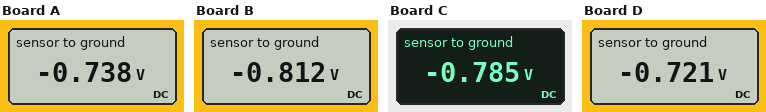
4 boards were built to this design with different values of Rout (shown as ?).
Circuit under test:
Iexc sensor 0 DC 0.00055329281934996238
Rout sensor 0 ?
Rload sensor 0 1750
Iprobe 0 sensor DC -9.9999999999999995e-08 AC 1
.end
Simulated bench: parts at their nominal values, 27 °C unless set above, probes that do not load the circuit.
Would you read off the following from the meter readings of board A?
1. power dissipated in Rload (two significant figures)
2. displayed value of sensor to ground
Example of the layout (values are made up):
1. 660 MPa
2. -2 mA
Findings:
1. 310 µW
2. -0.738 V
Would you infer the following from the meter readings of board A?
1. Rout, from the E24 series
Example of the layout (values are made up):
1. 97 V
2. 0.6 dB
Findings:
1. 5.6 kΩ
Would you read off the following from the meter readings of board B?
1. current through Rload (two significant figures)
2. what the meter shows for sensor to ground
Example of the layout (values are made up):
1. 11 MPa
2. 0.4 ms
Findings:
1. 460 µA
2. -0.812 V
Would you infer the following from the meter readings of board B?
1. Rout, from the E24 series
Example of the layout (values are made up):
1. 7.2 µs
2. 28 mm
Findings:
1. 9.1 kΩ
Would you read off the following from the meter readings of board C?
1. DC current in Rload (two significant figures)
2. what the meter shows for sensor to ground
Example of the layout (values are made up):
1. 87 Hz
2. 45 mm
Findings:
1. 450 µA
2. -0.785 V
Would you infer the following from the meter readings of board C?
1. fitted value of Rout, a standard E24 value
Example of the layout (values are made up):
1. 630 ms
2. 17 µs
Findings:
1. 7.5 kΩ
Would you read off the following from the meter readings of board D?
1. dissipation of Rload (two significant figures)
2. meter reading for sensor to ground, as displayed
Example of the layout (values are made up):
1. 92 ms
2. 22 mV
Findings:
1. 300 µW
2. -0.721 V
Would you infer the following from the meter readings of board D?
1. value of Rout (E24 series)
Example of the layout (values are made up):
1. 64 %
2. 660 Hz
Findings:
1. 5.1 kΩ
